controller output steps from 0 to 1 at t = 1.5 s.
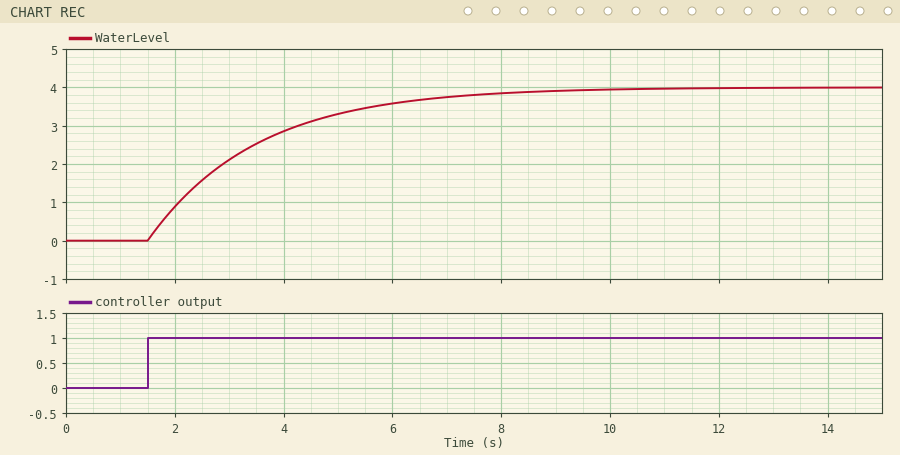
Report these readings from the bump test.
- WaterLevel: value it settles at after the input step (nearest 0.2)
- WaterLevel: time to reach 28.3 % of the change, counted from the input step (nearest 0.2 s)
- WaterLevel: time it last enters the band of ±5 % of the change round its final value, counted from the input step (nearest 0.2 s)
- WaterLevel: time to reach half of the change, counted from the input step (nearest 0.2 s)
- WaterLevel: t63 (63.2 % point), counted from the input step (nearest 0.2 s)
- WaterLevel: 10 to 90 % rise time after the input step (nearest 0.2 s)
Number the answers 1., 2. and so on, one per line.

1. 4.0
2. 0.6 s
3. 6.0 s
4. 1.4 s
5. 2.0 s
6. 4.4 s
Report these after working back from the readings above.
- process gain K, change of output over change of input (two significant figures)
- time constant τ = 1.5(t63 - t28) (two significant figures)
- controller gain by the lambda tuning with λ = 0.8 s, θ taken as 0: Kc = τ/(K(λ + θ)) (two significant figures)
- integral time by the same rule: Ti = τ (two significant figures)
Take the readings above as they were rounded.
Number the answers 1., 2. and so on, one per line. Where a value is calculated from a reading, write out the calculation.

1. (4 - 0) / 1 = 4.0
2. 1.5 × (2 - 0.6) = 2.1 s
3. 2.1 / (4 × (0.8 + 0)) = 0.66
4. 2.1 s
